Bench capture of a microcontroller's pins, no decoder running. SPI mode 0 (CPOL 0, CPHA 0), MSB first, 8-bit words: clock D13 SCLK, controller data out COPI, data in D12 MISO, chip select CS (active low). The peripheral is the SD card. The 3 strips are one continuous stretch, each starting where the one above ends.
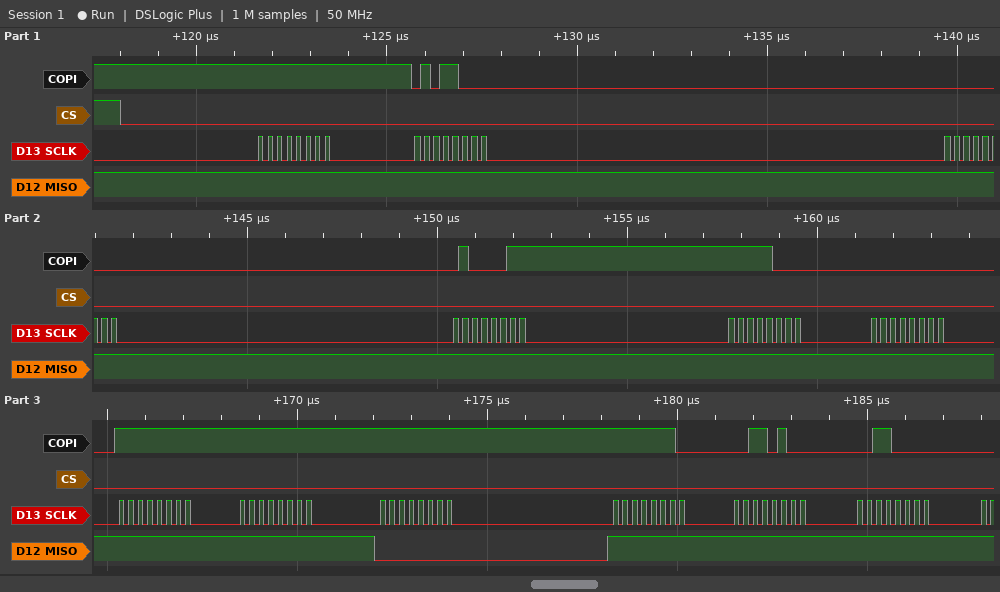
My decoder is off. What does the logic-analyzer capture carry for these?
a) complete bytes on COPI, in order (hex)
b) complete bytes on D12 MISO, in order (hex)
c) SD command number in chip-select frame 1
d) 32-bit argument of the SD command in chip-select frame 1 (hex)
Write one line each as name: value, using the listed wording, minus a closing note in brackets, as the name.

complete bytes on COPI, in order: FF 58 00 43 F8 00 FF FF FF FE 34 30
complete bytes on D12 MISO, in order: FF FF FF FF FF FF FF FF 00 FF FF FF
SD command number in chip-select frame 1: CMD24
32-bit argument of the SD command in chip-select frame 1: 0x0043F800
